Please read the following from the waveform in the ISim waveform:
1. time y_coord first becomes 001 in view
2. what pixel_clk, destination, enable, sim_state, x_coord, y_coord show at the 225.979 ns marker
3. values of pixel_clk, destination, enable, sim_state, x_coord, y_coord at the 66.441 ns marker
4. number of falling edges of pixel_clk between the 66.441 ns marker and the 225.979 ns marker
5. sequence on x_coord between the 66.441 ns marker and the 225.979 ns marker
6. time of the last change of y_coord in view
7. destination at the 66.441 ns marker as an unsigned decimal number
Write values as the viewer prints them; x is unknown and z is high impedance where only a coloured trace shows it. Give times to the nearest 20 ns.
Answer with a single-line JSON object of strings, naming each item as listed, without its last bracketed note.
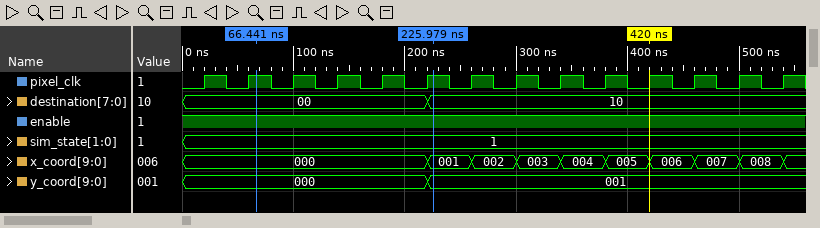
{"time y_coord first becomes 001 in view": "220 ns", "what pixel_clk, destination, enable, sim_state, x_coord, y_coord show at the 225.979 ns marker": "pixel_clk=1, destination=10, enable=1, sim_state=1, x_coord=001, y_coord=001", "values of pixel_clk, destination, enable, sim_state, x_coord, y_coord at the 66.441 ns marker": "pixel_clk=1, destination=00, enable=1, sim_state=1, x_coord=000, y_coord=000", "number of falling edges of pixel_clk between the 66.441 ns marker and the 225.979 ns marker": "4", "sequence on x_coord between the 66.441 ns marker and the 225.979 ns marker": "000, 001", "time of the last change of y_coord in view": "220 ns", "destination at the 66.441 ns marker as an unsigned decimal number": "0"}
